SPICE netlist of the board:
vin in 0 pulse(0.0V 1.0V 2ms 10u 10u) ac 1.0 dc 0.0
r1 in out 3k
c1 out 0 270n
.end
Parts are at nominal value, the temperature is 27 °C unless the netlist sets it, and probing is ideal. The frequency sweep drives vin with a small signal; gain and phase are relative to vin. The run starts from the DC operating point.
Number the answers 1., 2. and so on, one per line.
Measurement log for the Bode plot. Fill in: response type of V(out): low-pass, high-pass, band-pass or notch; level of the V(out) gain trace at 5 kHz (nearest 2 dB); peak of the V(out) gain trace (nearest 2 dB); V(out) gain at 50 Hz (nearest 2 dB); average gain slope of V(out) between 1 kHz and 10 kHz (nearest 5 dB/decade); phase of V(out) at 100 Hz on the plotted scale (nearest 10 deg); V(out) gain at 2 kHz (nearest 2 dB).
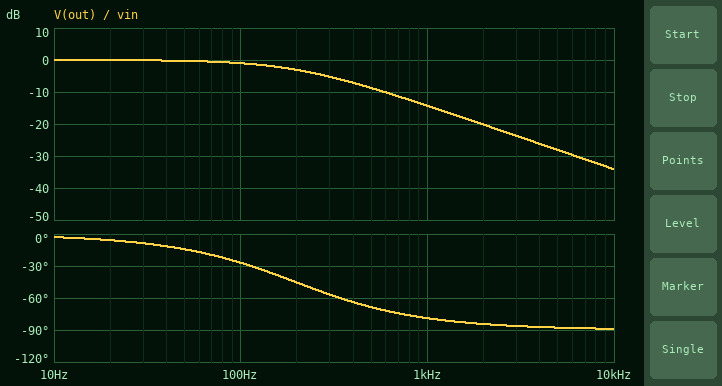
1. low-pass
2. -28 dB
3. 0 dB
4. 0 dB
5. -20 dB/decade
6. -30 deg
7. -20 dB
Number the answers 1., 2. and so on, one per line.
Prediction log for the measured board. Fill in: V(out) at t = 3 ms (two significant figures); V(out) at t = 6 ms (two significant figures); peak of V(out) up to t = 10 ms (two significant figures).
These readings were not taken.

1. 710 mV
2. 990 mV
3. 1.0 V
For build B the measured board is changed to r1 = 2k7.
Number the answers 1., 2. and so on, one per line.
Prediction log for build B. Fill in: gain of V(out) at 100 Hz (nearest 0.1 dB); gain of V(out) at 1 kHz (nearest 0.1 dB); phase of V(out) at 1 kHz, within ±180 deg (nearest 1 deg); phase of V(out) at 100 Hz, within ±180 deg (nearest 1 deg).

1. -0.8 dB
2. -13.4 dB
3. -78 deg
4. -25 deg
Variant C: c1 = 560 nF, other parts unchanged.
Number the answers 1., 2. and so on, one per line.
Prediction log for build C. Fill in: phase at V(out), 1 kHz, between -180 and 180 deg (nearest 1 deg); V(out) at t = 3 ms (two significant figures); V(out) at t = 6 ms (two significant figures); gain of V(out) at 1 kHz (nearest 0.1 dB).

1. -85 deg
2. 450 mV
3. 910 mV
4. -20.5 dB
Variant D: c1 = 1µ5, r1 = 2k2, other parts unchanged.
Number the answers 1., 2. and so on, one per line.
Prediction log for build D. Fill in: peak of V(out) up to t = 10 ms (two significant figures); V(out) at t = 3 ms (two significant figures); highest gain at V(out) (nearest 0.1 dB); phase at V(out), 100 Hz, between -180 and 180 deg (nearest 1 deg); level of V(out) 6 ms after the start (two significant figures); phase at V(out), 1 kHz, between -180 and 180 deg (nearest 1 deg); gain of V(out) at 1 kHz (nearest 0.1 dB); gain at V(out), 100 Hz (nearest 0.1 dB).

1. 910 mV
2. 260 mV
3. 0 dB
4. -64 deg
5. 700 mV
6. -87 deg
7. -26.3 dB
8. -7.2 dB
